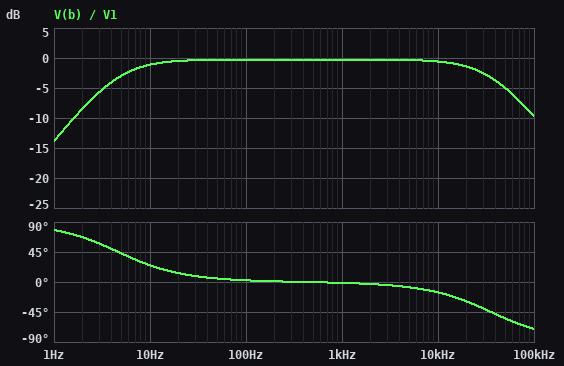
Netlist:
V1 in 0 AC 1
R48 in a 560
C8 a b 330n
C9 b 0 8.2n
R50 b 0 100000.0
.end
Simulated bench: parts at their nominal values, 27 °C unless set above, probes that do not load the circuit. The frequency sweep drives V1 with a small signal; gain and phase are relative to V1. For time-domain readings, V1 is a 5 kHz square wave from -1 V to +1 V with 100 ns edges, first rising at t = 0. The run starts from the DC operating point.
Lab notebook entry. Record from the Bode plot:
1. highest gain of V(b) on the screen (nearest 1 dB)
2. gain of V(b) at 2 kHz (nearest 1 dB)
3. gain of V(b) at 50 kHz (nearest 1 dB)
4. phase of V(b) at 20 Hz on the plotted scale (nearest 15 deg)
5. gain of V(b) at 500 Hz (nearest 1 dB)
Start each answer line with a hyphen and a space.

- 0 dB
- 0 dB
- -5 dB
- 15 deg
- 0 dB
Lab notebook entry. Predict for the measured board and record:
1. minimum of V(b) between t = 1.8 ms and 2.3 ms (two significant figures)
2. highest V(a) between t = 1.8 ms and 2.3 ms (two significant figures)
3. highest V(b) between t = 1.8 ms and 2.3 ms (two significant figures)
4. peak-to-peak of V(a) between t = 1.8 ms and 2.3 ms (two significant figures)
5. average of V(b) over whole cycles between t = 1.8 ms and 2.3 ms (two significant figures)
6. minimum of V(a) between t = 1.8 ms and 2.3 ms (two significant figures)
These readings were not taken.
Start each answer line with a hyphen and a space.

- -61 mV
- 990 mV
- 1.9 V
- 2.0 V
- 910 mV
- -1.0 V
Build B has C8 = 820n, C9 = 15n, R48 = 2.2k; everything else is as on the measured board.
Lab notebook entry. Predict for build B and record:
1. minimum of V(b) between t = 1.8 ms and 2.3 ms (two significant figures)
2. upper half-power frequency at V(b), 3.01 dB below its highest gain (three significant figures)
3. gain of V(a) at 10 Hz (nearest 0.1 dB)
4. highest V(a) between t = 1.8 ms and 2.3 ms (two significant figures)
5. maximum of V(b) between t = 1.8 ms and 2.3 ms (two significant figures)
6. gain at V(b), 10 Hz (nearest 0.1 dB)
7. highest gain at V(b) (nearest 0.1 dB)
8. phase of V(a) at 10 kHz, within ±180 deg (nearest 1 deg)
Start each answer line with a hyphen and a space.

- 55 mV
- 5.02 kHz
- -0.2 dB
- 880 mV
- 1.8 V
- -0.5 dB
- -0.3 dB
- -63 deg
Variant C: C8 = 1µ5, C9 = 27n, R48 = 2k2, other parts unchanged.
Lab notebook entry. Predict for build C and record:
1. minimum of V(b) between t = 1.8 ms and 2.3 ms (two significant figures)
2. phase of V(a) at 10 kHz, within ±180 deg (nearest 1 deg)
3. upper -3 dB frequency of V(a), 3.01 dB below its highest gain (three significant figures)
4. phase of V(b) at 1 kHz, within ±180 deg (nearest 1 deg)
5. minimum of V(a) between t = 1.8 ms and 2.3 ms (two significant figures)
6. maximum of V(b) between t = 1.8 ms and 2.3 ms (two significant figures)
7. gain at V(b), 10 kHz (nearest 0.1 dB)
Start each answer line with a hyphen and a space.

- 270 mV
- -74 deg
- 2.67 kHz
- -20 deg
- -710 mV
- 1.6 V
- -11.8 dB
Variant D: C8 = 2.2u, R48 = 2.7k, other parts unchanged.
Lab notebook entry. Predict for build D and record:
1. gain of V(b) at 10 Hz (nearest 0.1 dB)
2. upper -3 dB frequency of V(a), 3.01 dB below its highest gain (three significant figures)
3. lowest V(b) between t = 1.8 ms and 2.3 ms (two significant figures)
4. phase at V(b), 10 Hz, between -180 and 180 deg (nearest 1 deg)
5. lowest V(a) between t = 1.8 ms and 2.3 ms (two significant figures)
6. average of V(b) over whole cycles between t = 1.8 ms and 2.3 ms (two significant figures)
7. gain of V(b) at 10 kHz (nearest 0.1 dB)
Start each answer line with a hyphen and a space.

- -0.3 dB
- 7.02 kHz
- 9.0 mV
- 4 deg
- -980 mV
- 960 mV
- -4.8 dB
